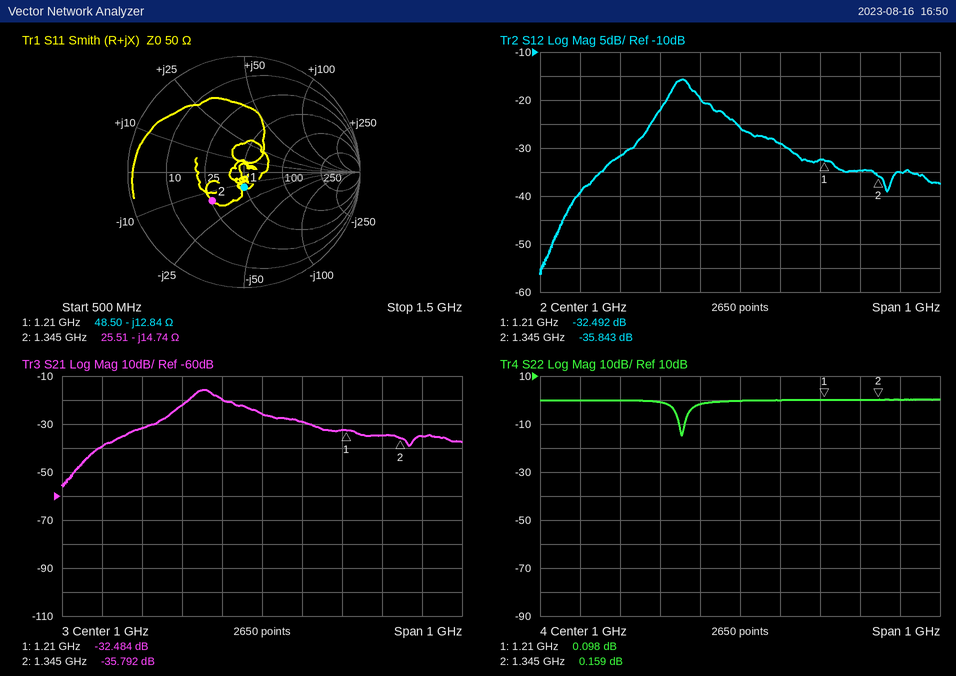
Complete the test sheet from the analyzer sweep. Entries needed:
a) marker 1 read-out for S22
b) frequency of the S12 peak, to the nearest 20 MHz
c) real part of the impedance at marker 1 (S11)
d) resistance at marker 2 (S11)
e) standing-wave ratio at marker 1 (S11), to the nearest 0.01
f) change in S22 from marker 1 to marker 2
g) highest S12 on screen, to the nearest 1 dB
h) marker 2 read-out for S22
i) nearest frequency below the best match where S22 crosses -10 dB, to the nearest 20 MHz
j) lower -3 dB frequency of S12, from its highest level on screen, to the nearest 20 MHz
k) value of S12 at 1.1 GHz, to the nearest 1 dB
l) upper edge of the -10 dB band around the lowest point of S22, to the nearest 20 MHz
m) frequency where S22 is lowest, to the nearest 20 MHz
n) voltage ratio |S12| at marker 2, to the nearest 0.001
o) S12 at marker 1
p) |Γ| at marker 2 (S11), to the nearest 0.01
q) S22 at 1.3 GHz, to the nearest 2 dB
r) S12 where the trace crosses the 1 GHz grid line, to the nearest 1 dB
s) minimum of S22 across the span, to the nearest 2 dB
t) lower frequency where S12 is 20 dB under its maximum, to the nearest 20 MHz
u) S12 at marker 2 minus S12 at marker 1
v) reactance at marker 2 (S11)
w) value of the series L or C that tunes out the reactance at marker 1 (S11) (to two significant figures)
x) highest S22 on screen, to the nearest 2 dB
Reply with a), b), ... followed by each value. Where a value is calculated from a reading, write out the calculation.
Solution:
a) 0.098 dB
b) 860 MHz
c) 48.50 Ω
d) 25.51 Ω
e) 1.30
f) 0.159 − (0.098) = 0.061 dB
g) -16 dB
h) 0.159 dB
i) 840 MHz
j) 820 MHz
k) -29 dB
l) 860 MHz
m) 860 MHz
n) 10^(-35.843/20) ≈ 0.016
o) -32.492 dB
p) 0.37
q) 0 dB
r) -26 dB
s) -14 dB
t) 640 MHz
u) -35.843 − (-32.492) = -3.351 dB
v) -14.74 Ω
w) L = 12.84 Ω/(2π × 1.21 GHz) ≈ 1.7 nH
x) 0 dB
